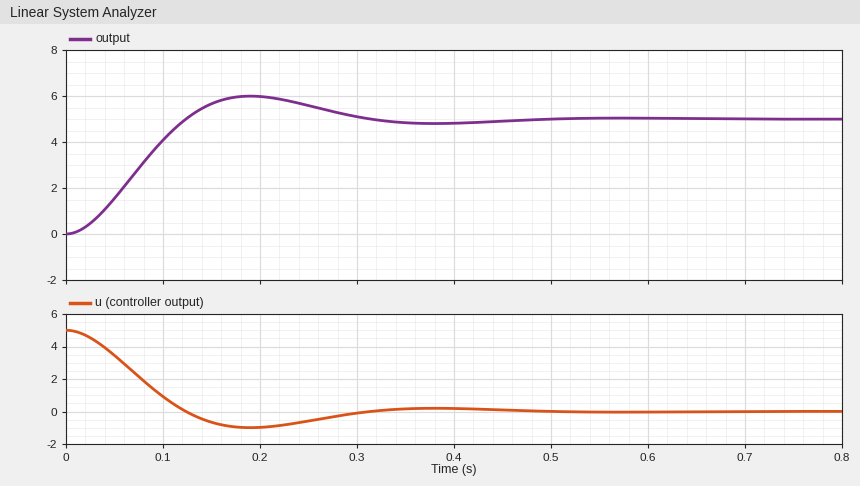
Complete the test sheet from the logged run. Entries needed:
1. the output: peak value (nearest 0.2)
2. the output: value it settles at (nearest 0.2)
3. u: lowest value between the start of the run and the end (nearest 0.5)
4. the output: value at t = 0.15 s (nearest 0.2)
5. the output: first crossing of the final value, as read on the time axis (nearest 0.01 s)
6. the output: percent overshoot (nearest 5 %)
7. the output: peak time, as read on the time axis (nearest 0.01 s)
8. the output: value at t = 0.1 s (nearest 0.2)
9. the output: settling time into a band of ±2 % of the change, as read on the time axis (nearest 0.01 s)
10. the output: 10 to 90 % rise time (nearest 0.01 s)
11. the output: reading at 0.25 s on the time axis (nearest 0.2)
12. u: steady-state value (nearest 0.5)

6.0
5.0
-1.0
5.6
0.12 s
20 %
0.19 s
4.0
0.45 s
0.08 s
5.6
0.0
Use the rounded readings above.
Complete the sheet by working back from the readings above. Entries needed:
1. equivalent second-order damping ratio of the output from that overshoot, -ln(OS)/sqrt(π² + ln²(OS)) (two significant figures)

0.46
